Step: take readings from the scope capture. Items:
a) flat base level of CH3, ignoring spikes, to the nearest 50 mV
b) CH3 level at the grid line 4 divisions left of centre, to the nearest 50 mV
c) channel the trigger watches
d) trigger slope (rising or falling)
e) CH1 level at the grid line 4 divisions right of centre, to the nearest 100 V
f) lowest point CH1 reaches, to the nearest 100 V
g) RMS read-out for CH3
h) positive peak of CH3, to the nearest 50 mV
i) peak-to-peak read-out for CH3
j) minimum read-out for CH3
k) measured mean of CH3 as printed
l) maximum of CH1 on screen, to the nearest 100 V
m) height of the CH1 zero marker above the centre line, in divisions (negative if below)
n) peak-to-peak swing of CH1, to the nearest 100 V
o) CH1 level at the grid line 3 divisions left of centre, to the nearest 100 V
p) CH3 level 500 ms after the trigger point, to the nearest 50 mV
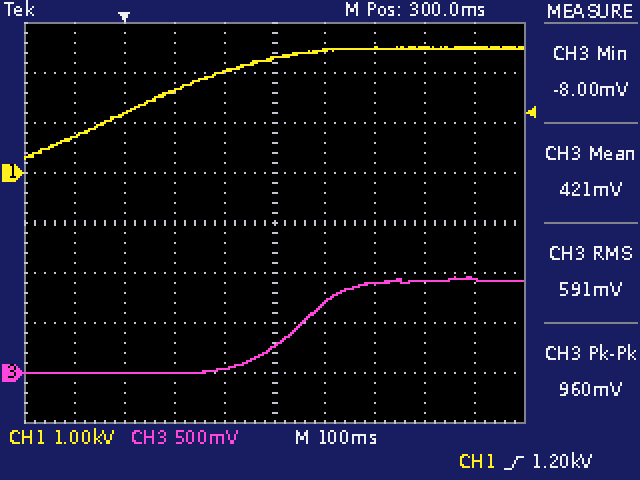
0 mV
0 mV
CH1
rising
2.5 kV
300 V
591 mV
950 mV
960 mV
-8.00 mV
421 mV
2.5 kV
+1.0 div
2.2 kV
1.2 kV
900 mV
